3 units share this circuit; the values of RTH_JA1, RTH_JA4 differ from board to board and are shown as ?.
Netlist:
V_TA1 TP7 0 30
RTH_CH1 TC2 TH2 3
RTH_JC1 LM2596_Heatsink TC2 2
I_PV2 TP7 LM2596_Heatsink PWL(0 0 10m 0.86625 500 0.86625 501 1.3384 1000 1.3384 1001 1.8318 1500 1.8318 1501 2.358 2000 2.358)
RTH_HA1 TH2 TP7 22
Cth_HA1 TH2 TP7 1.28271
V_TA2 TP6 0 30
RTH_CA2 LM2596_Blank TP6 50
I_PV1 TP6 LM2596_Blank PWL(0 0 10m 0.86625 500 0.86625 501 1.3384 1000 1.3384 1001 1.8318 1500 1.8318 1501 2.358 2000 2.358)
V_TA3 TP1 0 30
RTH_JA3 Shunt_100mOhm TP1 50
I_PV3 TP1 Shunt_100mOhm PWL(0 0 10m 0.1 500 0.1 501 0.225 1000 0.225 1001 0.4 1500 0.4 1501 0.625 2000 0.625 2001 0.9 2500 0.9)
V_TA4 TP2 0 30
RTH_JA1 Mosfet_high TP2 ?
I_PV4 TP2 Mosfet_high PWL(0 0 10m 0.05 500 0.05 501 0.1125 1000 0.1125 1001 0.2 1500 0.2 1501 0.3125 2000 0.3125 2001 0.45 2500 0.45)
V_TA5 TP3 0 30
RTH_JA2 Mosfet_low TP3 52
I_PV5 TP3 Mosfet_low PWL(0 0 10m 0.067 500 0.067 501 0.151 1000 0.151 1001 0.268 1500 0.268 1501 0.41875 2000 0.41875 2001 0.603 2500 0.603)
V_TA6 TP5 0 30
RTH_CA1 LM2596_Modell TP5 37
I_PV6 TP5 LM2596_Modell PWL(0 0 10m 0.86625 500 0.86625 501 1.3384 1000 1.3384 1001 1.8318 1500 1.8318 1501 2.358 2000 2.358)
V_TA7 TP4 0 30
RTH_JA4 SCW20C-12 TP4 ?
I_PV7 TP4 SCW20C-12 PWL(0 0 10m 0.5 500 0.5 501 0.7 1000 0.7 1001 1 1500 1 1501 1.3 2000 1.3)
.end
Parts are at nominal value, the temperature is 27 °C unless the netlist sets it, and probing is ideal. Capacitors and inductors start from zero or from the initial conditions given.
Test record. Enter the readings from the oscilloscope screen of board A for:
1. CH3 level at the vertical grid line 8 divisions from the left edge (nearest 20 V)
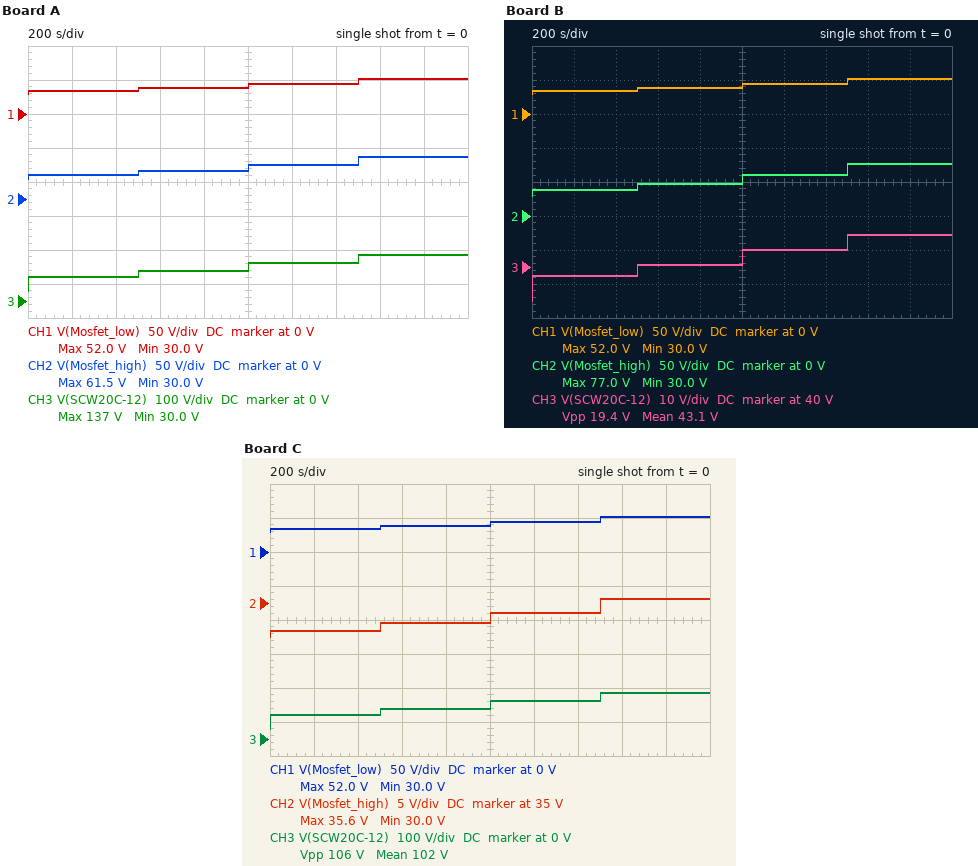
140 V
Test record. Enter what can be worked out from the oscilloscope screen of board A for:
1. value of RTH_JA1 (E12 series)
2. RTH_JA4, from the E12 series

100 Ω
82 Ω
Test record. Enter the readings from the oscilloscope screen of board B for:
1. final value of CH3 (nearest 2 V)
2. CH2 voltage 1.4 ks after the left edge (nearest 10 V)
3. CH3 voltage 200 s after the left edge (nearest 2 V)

50 V
60 V
38 V
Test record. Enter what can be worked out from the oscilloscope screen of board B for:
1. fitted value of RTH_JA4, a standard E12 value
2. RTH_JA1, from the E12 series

15 Ω
150 Ω
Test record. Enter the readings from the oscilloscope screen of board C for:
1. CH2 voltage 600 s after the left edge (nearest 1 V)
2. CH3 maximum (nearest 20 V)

32 V
140 V
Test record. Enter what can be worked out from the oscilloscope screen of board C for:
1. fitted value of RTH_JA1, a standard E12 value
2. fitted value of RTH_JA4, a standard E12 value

18 Ω
82 Ω
